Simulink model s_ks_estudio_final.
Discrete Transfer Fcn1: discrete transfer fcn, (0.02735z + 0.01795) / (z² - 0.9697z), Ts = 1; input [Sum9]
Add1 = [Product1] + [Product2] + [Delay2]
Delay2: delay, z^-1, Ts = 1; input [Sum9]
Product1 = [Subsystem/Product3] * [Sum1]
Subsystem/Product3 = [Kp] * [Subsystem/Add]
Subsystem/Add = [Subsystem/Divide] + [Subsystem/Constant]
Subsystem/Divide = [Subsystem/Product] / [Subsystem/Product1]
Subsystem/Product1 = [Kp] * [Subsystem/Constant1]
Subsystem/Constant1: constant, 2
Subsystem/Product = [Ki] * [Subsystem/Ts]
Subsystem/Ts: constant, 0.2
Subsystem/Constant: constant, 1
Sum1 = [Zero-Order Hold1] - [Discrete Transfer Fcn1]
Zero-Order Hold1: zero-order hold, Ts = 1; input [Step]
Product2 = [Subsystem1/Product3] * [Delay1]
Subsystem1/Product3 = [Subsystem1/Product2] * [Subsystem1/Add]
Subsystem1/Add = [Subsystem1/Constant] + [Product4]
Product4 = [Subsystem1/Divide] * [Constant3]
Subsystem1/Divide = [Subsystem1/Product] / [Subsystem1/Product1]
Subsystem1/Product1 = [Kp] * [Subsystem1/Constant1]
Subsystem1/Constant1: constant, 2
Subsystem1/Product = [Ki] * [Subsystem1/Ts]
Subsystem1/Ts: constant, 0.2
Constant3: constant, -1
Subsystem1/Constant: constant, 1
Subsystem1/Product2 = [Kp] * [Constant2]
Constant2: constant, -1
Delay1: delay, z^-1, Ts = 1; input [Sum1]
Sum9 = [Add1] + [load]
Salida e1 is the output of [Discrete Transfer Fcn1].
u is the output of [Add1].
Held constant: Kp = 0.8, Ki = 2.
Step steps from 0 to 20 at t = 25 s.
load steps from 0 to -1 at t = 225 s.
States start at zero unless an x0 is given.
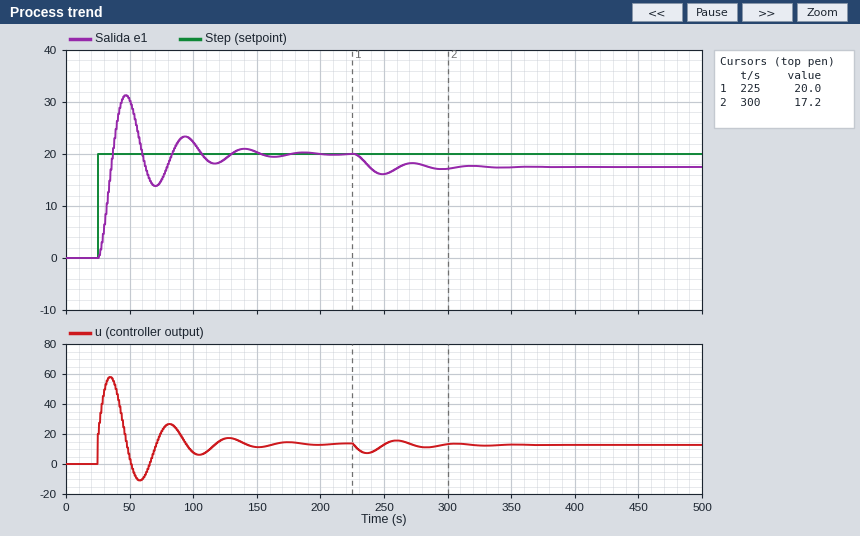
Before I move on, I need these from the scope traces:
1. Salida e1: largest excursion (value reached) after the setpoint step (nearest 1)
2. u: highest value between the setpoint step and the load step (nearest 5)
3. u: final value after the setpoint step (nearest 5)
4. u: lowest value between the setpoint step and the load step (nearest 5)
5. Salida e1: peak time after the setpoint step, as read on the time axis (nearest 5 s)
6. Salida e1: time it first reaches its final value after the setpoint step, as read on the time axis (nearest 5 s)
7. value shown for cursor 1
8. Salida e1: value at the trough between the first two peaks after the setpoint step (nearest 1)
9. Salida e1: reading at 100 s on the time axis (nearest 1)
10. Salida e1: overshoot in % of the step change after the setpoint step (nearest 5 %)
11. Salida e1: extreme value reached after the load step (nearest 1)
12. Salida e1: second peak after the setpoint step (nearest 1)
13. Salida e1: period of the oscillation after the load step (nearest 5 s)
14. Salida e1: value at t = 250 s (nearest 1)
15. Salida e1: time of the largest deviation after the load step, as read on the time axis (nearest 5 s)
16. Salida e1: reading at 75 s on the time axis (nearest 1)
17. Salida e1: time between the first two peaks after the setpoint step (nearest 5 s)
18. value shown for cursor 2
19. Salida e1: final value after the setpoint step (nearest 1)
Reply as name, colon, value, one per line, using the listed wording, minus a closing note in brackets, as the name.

Salida e1: largest excursion (value reached) after the setpoint step: 31
u: highest value between the setpoint step and the load step: 60
u: final value after the setpoint step: 15
u: lowest value between the setpoint step and the load step: -10
Salida e1: peak time after the setpoint step, as read on the time axis: 45 s
Salida e1: time it first reaches its final value after the setpoint step, as read on the time axis: 35 s
value shown for cursor 1: 20.0
Salida e1: value at the trough between the first two peaks after the setpoint step: 14
Salida e1: reading at 100 s on the time axis: 22
Salida e1: overshoot in % of the step change after the setpoint step: 55 %
Salida e1: extreme value reached after the load step: 16
Salida e1: second peak after the setpoint step: 23
Salida e1: period of the oscillation after the load step: 45 s
Salida e1: value at t = 250 s: 16
Salida e1: time of the largest deviation after the load step, as read on the time axis: 250 s
Salida e1: reading at 75 s on the time axis: 15
Salida e1: time between the first two peaks after the setpoint step: 45 s
value shown for cursor 2: 17.2
Salida e1: final value after the setpoint step: 20
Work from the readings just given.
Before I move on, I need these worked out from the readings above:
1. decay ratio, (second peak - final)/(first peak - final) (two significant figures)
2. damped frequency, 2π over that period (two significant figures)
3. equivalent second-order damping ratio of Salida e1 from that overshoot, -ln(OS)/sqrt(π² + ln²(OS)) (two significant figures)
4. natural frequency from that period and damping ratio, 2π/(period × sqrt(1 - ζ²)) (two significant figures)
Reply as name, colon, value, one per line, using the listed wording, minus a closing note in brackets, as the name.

decay ratio, (second peak - final)/(first peak - final): 0.27
damped frequency, 2π over that period: 0.14 rad/s
equivalent second-order damping ratio of Salida e1 from that overshoot, -ln(OS)/sqrt(π² + ln²(OS)): 0.19
natural frequency from that period and damping ratio, 2π/(period × sqrt(1 - ζ²)): 0.14 rad/s
